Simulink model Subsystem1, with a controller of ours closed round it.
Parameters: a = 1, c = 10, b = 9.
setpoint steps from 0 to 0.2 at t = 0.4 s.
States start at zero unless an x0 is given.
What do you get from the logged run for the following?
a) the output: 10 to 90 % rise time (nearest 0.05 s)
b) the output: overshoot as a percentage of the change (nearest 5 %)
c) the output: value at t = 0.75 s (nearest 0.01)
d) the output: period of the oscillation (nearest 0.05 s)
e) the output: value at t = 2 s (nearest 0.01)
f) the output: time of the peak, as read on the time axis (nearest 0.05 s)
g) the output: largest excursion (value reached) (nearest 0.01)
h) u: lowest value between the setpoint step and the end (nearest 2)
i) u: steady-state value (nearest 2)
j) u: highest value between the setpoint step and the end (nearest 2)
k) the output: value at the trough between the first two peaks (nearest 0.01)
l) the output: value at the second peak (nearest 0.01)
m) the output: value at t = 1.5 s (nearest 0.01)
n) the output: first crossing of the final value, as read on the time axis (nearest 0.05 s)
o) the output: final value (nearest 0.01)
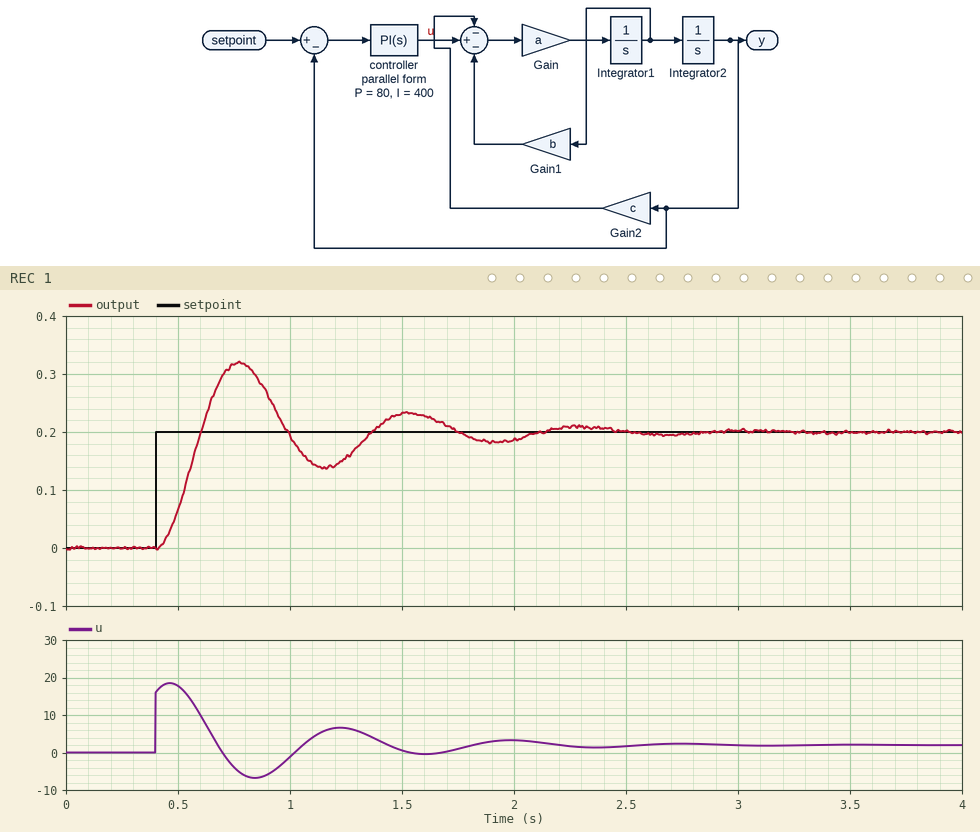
0.15 s
60 %
0.32
0.75 s
0.19
0.75 s
0.32
-6
2
18
0.14
0.23
0.23
0.60 s
0.20
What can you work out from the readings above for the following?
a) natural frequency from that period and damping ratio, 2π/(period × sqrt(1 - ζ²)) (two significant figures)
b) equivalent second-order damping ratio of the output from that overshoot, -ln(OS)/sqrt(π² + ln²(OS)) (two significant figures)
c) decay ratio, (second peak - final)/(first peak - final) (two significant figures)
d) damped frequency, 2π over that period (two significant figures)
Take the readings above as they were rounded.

8.5 rad/s
0.16
0.25
8.4 rad/s
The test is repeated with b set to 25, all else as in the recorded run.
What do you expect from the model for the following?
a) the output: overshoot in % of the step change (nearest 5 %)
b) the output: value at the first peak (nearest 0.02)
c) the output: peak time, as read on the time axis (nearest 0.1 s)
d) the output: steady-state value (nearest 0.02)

40 %
0.28
1.0 s
0.20
